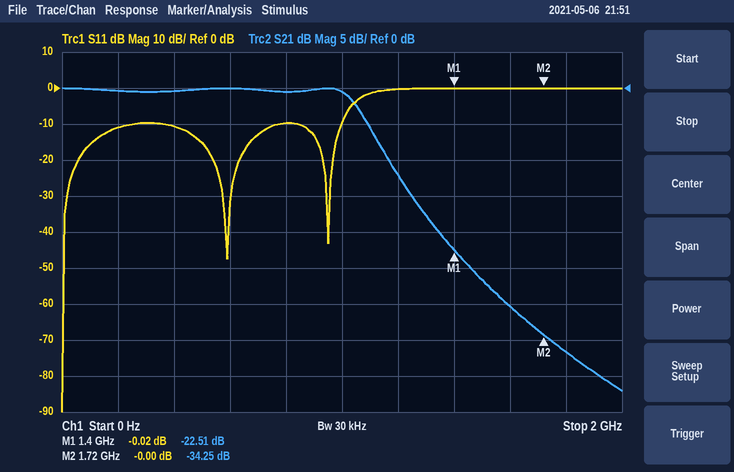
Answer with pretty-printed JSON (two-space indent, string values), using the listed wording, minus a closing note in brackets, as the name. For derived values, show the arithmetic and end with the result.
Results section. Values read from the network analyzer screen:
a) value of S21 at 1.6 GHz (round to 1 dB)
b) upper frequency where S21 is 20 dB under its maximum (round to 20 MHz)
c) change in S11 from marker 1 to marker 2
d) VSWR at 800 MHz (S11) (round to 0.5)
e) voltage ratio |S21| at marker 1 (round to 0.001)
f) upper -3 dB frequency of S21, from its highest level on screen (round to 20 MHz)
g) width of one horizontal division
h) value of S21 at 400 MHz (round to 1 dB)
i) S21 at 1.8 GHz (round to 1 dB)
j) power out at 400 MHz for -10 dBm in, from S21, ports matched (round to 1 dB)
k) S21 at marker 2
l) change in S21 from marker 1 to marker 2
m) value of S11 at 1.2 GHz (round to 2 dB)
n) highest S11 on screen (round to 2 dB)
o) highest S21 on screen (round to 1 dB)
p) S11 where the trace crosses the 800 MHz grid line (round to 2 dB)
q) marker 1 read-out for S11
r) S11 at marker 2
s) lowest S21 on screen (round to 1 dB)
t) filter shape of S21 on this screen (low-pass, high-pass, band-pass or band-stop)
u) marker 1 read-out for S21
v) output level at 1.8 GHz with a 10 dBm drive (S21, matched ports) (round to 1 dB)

{
  "value of S21 at 1.6 GHz": "-30 dB",
  "upper frequency where S21 is 20 dB under its maximum": "1.34 GHz",
  "change in S11 from marker 1 to marker 2": "-0 − (-0.02) = 0.02 dB",
  "VSWR at 800 MHz (S11)": "|Γ| = 10^(-10/20) = 0.3162; VSWR = (1 + 0.3162)/(1 − 0.3162) ≈ 1.92, so 2.0 to the nearest 0.5",
  "voltage ratio |S21| at marker 1": "10^(-22.51/20) ≈ 0.075",
  "upper -3 dB frequency of S21, from its highest level on screen": "1.06 GHz",
  "width of one horizontal division": "200 MHz",
  "value of S21 at 400 MHz": "0 dB",
  "S21 at 1.8 GHz": "-37 dB",
  "power out at 400 MHz for -10 dBm in, from S21, ports matched": "-10 dBm + (0 dB) = -10 dBm",
  "S21 at marker 2": "-34.25 dB",
  "change in S21 from marker 1 to marker 2": "-34.25 − (-22.51) = -11.74 dB",
  "value of S11 at 1.2 GHz": "0 dB",
  "highest S11 on screen": "0 dB",
  "highest S21 on screen": "0 dB",
  "S11 where the trace crosses the 800 MHz grid line": "-10 dB",
  "marker 1 read-out for S11": "-0.02 dB",
  "S11 at marker 2": "-0.00 dB",
  "lowest S21 on screen": "-42 dB",
  "filter shape of S21 on this screen": "low-pass",
  "marker 1 read-out for S21": "-22.51 dB",
  "output level at 1.8 GHz with a 10 dBm drive (S21, matched ports)": "10 dBm + (-37 dB) = -27 dBm"
}
